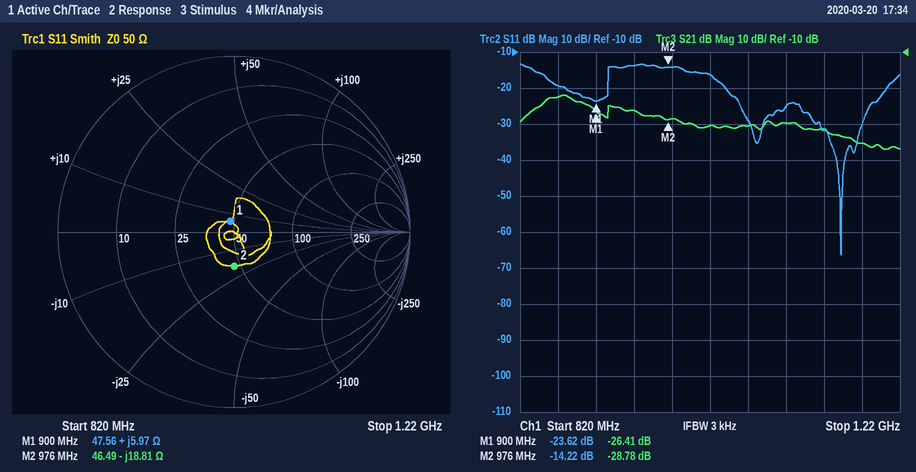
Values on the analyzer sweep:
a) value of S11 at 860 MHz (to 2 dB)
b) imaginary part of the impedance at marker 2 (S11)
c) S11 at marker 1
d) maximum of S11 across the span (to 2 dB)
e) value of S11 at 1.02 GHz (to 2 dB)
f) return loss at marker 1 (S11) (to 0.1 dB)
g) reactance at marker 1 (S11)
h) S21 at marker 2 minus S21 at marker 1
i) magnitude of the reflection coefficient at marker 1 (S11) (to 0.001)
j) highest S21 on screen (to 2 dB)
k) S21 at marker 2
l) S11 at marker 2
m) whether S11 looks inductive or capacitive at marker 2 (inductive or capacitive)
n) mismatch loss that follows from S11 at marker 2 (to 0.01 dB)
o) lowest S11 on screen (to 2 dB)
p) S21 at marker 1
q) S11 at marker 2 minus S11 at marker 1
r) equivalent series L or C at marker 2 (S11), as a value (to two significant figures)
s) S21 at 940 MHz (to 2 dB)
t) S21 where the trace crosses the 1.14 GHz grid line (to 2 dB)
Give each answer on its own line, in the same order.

-20 dB
-18.81 Ω
-23.62 dB
-14 dB
-16 dB
23.6 dB
+5.97 Ω
-2.37 dB
0.066
-22 dB
-28.78 dB
-14.22 dB
capacitive
0.17 dB
-66 dB
-26.41 dB
9.40 dB
8.7 pF
-26 dB
-32 dB
